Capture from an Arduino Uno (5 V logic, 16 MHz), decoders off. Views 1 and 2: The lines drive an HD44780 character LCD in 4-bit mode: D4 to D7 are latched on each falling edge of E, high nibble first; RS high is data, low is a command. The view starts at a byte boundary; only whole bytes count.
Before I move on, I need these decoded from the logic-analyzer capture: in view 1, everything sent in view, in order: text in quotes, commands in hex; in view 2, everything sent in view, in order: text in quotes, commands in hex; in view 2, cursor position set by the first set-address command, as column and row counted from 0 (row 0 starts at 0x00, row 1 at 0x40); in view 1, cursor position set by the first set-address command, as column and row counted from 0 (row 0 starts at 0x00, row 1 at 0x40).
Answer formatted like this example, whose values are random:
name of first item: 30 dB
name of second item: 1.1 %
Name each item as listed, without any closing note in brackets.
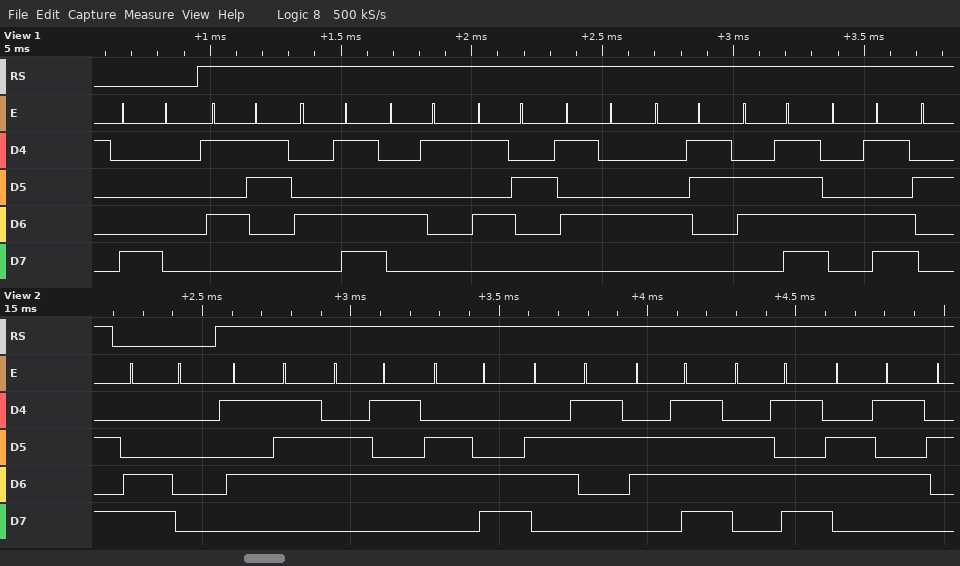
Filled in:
in view 1, everything sent in view, in order: text in quotes, commands in hex: 0x80 "SMARTCoM"
in view 2, everything sent in view, in order: text in quotes, commands in hex: 0xC0 "Welcome"
in view 2, cursor position set by the first set-address command, as column and row counted from 0: column 0, row 1
in view 1, cursor position set by the first set-address command, as column and row counted from 0: column 0, row 0
